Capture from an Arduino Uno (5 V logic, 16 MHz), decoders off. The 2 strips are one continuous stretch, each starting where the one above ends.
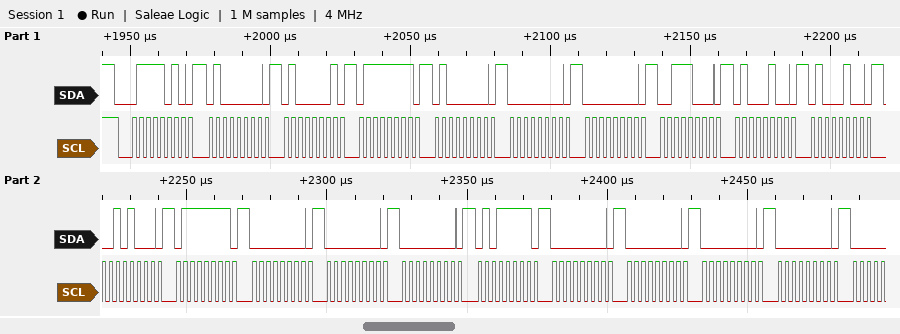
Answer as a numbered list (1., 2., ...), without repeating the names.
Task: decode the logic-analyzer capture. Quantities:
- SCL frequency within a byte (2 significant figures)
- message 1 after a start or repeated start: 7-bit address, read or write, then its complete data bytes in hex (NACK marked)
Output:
1. 400 kHz
2. 0x3D write: 40 41 7F 40 00 00 38 44 44 28 7F 00 00 00 5F 00 00 00 00
